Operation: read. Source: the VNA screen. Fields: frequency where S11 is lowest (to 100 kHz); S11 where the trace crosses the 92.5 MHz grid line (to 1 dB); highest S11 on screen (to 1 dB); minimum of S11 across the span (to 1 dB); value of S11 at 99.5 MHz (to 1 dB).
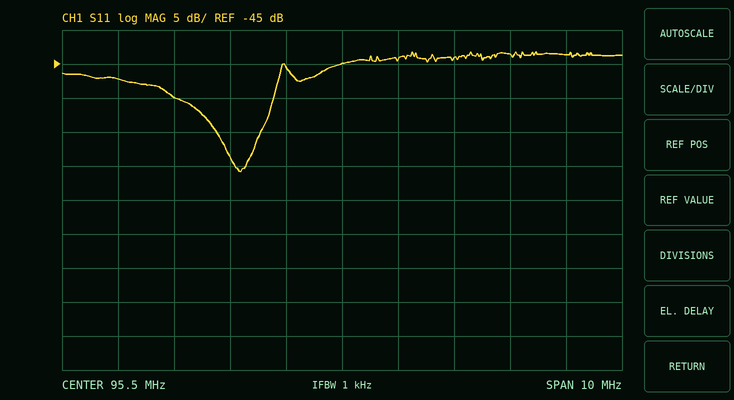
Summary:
93.7 MHz
-50 dB
-43 dB
-61 dB
-44 dB
